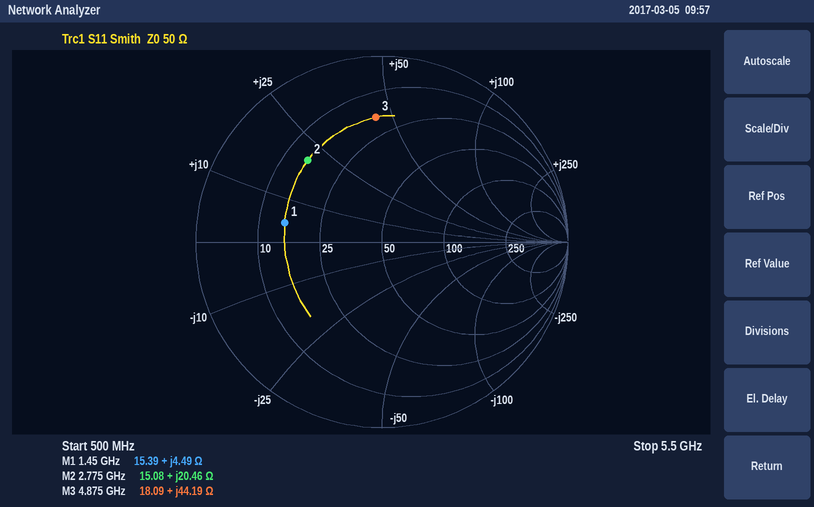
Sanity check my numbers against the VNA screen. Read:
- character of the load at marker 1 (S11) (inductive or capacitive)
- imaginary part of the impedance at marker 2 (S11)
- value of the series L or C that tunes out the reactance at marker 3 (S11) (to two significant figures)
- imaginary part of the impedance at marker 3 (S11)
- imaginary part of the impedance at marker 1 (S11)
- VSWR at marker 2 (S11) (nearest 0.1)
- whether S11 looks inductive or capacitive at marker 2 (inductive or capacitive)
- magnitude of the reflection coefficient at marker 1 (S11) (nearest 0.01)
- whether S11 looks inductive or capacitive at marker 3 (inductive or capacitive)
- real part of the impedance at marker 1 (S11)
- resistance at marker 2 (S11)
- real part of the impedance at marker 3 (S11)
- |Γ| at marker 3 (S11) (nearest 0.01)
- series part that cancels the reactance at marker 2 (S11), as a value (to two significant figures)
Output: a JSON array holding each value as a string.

["inductive", "+20.46 Ω", "740 fF", "+44.19 Ω", "+4.49 Ω", "3.9", "inductive", "0.53", "inductive", "15.39 Ω", "15.08 Ω", "18.09 Ω", "0.67", "2.8 pF"]
